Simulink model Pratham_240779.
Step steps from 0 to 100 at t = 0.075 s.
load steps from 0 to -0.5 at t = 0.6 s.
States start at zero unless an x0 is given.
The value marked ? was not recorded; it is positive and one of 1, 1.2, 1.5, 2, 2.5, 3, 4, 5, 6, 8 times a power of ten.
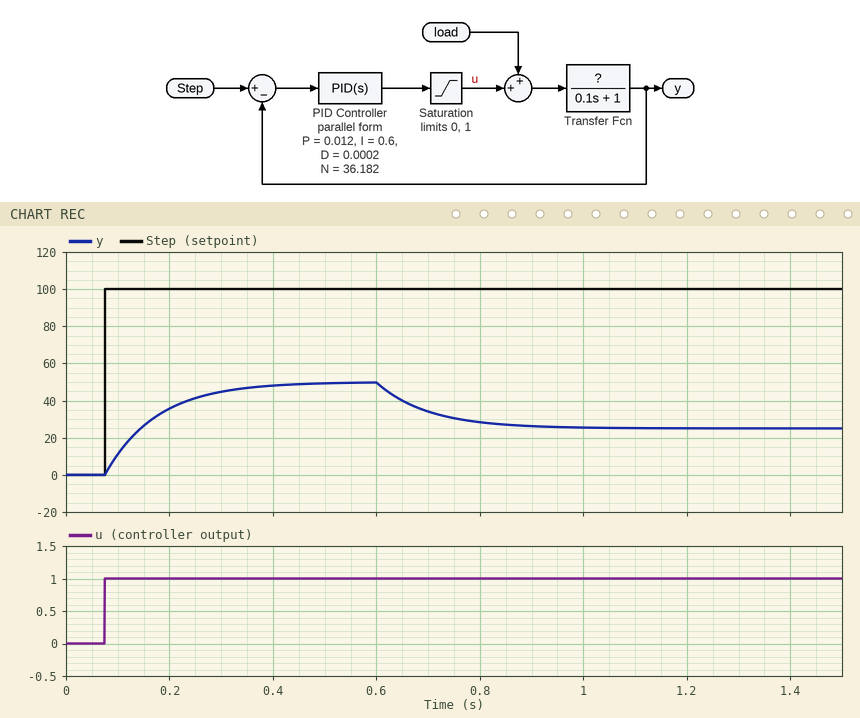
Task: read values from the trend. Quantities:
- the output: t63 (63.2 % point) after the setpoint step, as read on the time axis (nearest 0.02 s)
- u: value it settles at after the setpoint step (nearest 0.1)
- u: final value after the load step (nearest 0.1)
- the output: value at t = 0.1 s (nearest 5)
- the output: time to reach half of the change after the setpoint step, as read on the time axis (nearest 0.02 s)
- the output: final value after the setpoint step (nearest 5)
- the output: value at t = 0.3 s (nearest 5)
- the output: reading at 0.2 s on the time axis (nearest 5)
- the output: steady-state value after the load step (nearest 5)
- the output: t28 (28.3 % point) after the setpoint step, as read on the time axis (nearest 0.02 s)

0.18 s
1.0
1.0
10
0.14 s
50
45
35
25
0.10 s
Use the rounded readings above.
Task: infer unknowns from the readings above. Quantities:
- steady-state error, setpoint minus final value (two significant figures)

50
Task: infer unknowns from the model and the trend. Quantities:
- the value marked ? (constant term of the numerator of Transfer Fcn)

50
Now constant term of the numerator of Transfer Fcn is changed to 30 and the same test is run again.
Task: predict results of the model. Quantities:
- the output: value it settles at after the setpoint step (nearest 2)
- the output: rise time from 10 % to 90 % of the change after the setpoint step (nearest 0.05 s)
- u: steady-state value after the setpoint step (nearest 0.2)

30
0.20 s
1.0
